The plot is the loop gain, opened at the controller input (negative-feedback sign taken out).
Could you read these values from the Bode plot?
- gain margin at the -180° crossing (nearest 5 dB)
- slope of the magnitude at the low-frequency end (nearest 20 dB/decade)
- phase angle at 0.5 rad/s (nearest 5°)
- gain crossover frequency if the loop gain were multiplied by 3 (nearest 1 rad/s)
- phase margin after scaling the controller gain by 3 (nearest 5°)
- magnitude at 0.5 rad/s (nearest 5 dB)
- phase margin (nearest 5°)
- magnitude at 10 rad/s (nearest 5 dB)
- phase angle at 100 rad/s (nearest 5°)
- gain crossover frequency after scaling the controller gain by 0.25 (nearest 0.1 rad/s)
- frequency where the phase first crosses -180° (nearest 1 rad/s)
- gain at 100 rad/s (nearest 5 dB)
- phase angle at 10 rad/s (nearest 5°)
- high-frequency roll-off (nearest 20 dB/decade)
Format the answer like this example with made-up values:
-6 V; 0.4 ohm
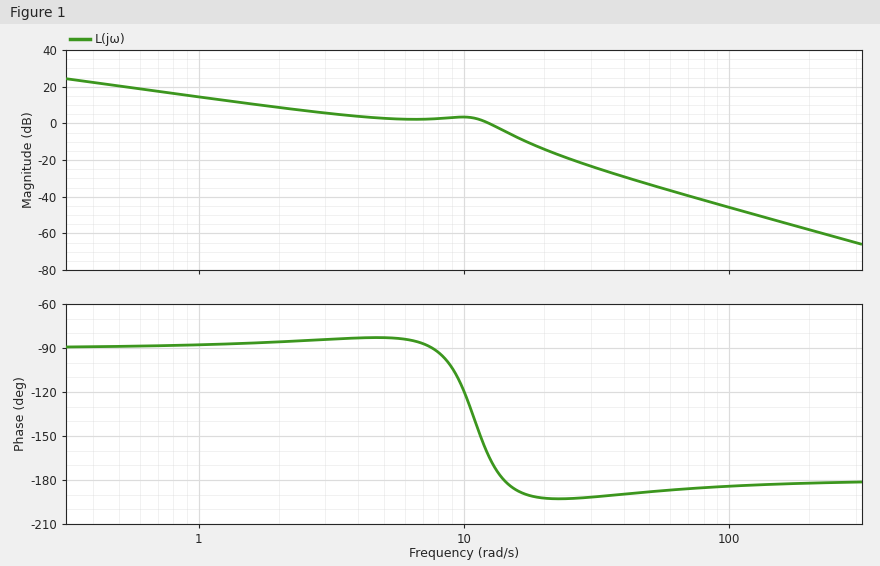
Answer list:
5 dB; -20 dB/decade; -90°; 17 rad/s; -10°; 20 dB; 15°; 5 dB; -185°; 1.3 rad/s; 14 rad/s; -45 dB; -120°; -40 dB/decade
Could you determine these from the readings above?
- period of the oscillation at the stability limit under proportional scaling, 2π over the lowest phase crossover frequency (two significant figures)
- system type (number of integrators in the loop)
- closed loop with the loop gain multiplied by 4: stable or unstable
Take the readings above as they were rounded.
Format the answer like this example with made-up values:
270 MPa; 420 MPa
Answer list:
0.45 s; 1; unstable
